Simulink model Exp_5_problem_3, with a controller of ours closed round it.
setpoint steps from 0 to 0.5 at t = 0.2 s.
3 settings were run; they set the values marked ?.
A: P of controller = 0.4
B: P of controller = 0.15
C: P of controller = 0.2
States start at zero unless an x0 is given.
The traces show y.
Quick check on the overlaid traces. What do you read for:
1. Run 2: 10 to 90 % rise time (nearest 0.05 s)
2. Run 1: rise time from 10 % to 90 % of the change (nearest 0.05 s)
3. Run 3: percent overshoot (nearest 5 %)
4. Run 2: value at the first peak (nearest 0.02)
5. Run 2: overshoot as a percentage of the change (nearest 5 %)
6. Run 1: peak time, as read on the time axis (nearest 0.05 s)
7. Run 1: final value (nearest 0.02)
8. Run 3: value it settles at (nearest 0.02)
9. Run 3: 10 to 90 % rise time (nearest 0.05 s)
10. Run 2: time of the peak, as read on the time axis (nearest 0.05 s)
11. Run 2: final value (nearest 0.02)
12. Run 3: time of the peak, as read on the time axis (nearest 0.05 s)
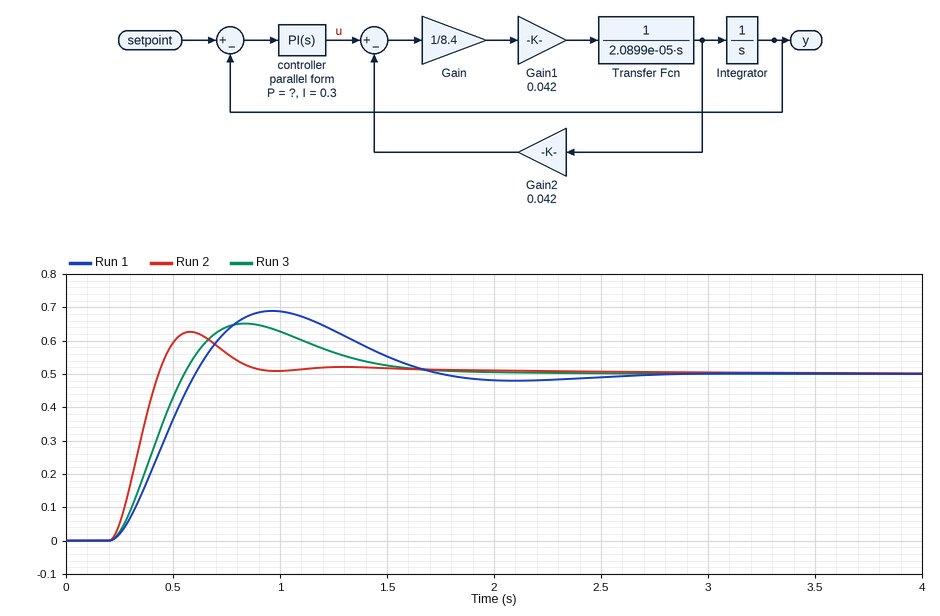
0.15 s
0.30 s
30 %
0.62
25 %
0.95 s
0.50
0.50
0.25 s
0.60 s
0.50
0.85 s
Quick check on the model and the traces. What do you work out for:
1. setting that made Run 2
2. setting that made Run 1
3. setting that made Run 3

A
B
C
